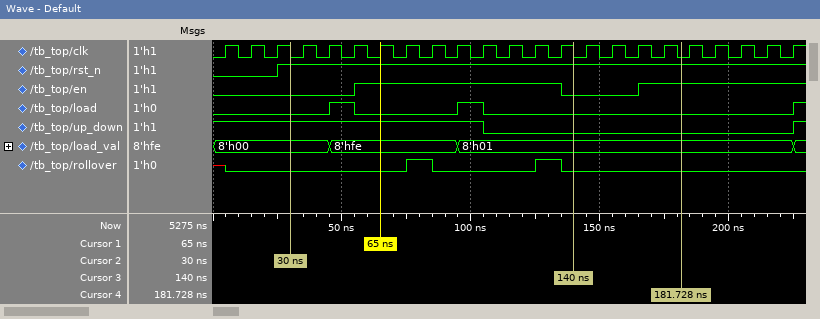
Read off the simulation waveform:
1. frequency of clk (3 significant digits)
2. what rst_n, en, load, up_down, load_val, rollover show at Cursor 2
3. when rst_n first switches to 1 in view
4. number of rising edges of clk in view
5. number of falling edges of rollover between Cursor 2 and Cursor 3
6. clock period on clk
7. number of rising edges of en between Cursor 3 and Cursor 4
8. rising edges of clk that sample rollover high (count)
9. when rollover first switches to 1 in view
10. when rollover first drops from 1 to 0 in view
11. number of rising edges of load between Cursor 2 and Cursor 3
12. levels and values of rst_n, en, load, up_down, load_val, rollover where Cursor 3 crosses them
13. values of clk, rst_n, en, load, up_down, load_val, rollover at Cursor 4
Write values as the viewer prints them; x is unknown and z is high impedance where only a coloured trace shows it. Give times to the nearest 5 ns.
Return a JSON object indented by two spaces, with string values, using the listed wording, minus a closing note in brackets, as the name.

{
  "frequency of clk": "100 MHz",
  "what rst_n, en, load, up_down, load_val, rollover show at Cursor 2": "rst_n=1, en=0, load=0, up_down=1, load_val=8'h00, rollover=0",
  "when rst_n first switches to 1 in view": "25 ns",
  "number of rising edges of clk in view": "23",
  "number of falling edges of rollover between Cursor 2 and Cursor 3": "2",
  "clock period on clk": "10 ns",
  "number of rising edges of en between Cursor 3 and Cursor 4": "1",
  "rising edges of clk that sample rollover high": "2",
  "when rollover first switches to 1 in view": "75 ns",
  "when rollover first drops from 1 to 0 in view": "85 ns",
  "number of rising edges of load between Cursor 2 and Cursor 3": "2",
  "levels and values of rst_n, en, load, up_down, load_val, rollover where Cursor 3 crosses them": "rst_n=1, en=0, load=0, up_down=0, load_val=8'h01, rollover=0",
  "values of clk, rst_n, en, load, up_down, load_val, rollover at Cursor 4": "clk=0, rst_n=1, en=1, load=0, up_down=0, load_val=8'h01, rollover=0"
}
